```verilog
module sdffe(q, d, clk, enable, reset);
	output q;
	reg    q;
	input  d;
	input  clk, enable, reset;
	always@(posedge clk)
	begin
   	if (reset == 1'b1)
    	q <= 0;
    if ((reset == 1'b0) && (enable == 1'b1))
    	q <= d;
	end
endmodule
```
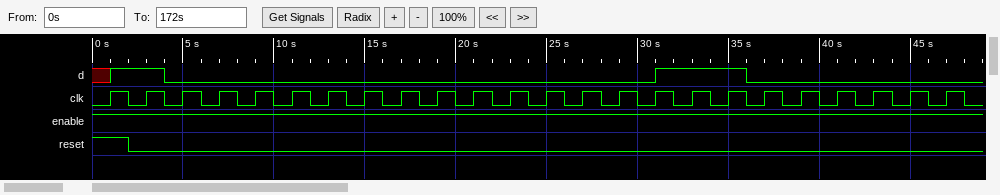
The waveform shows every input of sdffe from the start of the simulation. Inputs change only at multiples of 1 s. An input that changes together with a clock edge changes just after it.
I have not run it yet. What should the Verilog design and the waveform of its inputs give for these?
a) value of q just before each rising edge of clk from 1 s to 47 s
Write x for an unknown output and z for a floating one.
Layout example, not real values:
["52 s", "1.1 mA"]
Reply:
["x 0 1 0 0 0 0 0 0 0 0 0 0 0 0 0 0 1 1 0 0 0 0 0"]
